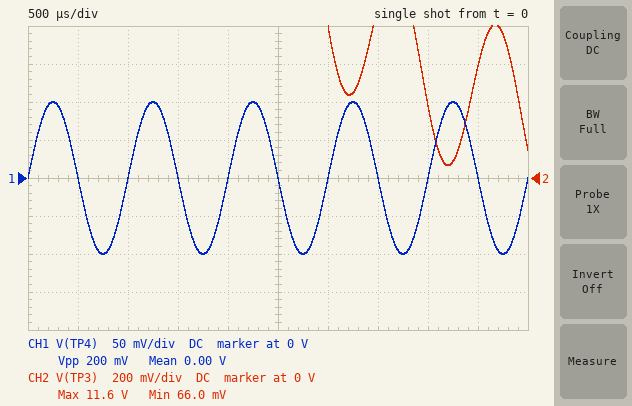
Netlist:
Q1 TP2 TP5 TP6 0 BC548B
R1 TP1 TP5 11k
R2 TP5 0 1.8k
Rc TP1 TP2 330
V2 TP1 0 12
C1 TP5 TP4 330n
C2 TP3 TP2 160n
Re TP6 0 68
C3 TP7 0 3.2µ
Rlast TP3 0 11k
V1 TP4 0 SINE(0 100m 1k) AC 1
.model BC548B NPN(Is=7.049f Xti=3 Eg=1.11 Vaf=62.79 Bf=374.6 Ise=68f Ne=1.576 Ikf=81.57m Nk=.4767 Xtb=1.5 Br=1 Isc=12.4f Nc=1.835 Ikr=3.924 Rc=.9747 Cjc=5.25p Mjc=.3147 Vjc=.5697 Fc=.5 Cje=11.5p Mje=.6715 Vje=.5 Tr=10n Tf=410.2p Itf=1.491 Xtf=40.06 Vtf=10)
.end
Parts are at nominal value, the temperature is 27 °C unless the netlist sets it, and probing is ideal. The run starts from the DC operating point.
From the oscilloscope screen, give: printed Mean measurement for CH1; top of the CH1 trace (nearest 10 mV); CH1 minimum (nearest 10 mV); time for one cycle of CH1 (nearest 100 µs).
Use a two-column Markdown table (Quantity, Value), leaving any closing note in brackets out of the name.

| Quantity | Value |
|---|---|
| printed Mean measurement for CH1 | 0.00 V |
| top of the CH1 trace | 100 mV |
| CH1 minimum | -100 mV |
| time for one cycle of CH1 | 1.0 ms |
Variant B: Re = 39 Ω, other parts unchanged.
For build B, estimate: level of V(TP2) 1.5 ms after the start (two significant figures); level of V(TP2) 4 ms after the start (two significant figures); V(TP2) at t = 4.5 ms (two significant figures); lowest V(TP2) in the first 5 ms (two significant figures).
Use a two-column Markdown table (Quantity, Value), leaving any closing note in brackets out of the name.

| Quantity | Value |
|---|---|
| level of V(TP2) 1.5 ms after the start | 5.7 V |
| level of V(TP2) 4 ms after the start | 4.8 V |
| V(TP2) at t = 4.5 ms | 5.3 V |
| lowest V(TP2) in the first 5 ms | 4.3 V |
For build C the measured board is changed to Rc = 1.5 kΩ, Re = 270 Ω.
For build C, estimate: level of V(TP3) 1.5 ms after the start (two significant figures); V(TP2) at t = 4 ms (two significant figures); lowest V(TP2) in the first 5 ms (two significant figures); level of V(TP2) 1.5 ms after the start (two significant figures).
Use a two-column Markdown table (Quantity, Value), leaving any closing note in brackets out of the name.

| Quantity | Value |
|---|---|
| level of V(TP3) 1.5 ms after the start | 2.3 V |
| V(TP2) at t = 4 ms | 6.4 V |
| lowest V(TP2) in the first 5 ms | 6.1 V |
| level of V(TP2) 1.5 ms after the start | 6.9 V |
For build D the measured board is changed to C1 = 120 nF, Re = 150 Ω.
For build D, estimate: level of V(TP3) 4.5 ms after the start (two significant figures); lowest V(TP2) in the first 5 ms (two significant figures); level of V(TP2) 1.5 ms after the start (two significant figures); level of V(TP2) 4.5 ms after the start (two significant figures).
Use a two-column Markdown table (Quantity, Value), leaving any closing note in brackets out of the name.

| Quantity | Value |
|---|---|
| level of V(TP3) 4.5 ms after the start | 880 mV |
| lowest V(TP2) in the first 5 ms | 9.6 V |
| level of V(TP2) 1.5 ms after the start | 9.9 V |
| level of V(TP2) 4.5 ms after the start | 10 V |
